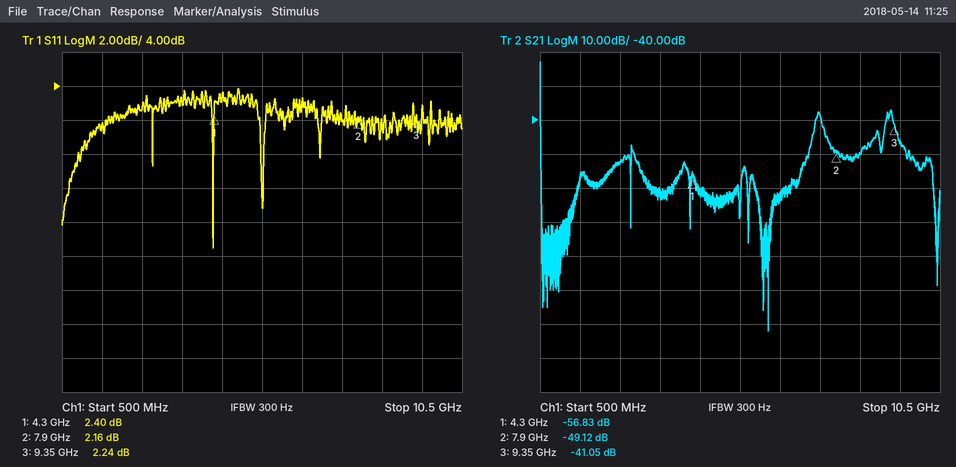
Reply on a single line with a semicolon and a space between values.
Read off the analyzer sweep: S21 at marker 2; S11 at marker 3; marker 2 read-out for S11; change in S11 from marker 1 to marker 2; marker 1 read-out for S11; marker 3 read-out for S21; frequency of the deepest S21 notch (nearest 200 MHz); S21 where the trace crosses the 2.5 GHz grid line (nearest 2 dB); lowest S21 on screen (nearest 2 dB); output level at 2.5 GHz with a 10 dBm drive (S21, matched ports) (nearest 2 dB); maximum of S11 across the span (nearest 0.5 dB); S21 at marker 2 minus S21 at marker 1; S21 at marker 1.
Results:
-49.12 dB; 2.24 dB; 2.16 dB; -0.24 dB; 2.40 dB; -41.05 dB; 6.2 GHz; -52 dB; -102 dB; -42 dBm; 4.0 dB; 7.71 dB; -56.83 dB
